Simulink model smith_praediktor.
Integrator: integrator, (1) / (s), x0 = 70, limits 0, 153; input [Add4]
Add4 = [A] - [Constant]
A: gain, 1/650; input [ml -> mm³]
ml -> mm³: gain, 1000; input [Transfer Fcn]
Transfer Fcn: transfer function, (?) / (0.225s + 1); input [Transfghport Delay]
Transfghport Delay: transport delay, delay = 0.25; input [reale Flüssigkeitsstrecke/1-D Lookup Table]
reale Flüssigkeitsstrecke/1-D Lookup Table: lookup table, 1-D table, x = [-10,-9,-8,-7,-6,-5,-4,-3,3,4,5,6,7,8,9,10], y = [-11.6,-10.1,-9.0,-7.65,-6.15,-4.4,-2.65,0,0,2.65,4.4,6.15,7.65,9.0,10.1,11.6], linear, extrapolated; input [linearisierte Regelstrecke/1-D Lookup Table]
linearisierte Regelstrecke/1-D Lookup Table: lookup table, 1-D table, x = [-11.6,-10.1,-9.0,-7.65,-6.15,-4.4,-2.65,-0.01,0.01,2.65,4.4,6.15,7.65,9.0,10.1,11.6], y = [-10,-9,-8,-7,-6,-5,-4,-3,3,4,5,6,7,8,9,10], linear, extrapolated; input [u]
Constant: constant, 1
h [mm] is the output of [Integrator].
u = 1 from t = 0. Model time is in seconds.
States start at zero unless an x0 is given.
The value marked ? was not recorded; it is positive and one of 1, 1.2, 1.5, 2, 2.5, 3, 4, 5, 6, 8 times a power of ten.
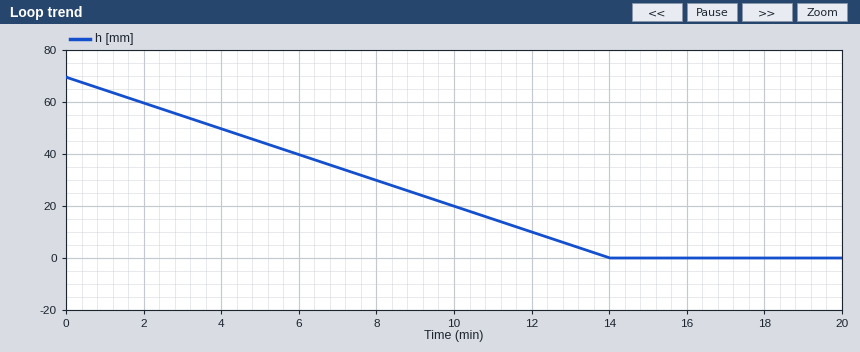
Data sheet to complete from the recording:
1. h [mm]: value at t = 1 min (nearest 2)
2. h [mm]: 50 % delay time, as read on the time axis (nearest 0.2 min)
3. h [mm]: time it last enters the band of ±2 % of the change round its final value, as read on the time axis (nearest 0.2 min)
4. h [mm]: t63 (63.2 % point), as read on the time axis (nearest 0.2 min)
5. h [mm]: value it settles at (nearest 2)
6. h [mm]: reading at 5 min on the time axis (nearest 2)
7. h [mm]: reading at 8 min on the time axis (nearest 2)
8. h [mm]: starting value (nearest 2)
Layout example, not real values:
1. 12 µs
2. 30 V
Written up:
1. 64
2. 7.0 min
3. 13.8 min
4. 8.8 min
5. 0
6. 44
7. 30
8. 70
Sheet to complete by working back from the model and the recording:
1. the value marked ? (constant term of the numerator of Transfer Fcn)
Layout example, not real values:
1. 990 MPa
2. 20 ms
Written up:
1. 0.6
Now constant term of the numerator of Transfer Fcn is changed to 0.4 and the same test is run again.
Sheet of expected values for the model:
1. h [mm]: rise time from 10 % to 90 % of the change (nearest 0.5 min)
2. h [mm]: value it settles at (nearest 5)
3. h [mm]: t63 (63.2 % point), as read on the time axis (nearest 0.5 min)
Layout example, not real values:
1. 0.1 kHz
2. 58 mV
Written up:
1. 2.5 min
2. 0
3. 2.0 min
